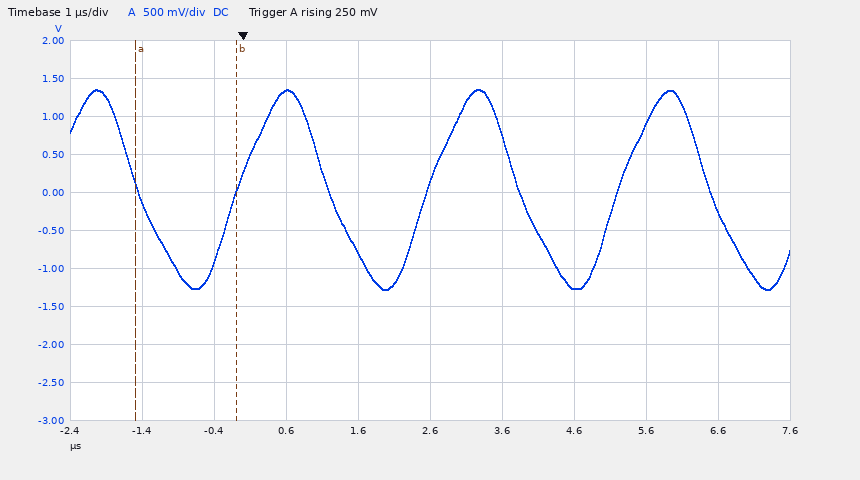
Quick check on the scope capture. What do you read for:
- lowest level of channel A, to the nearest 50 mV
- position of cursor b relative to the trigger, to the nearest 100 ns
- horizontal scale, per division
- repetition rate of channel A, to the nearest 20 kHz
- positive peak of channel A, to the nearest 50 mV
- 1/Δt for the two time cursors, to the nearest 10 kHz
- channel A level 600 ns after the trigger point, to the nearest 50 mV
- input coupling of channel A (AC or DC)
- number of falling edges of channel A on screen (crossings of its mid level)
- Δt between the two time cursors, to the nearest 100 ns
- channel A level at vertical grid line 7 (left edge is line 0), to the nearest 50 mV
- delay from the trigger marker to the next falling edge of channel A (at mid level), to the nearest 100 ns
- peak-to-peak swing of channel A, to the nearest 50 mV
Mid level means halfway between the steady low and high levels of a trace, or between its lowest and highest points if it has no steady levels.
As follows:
-1.30 V
-100 ns
1 µs
380 kHz
1.35 V
710 kHz
1.35 V
DC
4
1.4 µs
-1.25 V
1.2 µs
2.65 V
